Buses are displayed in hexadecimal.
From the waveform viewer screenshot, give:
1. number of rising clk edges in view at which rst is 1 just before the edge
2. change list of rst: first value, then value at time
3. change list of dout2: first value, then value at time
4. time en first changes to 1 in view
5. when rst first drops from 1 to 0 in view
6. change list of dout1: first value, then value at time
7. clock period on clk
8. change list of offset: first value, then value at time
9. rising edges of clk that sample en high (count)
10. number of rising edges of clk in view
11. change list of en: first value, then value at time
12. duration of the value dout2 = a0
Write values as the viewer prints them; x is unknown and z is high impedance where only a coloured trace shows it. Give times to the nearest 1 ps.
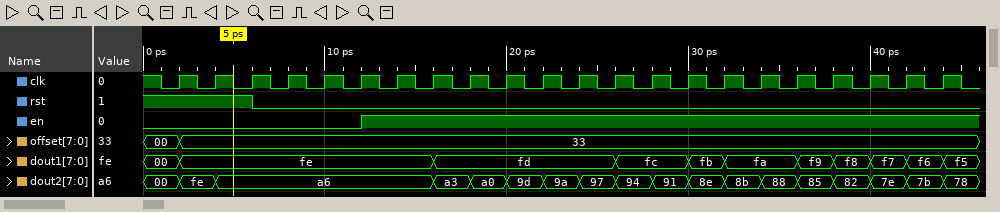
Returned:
3
1, 0 at 6 ps
00, fe at 2 ps, a6 at 4 ps, a3 at 16 ps, a0 at 18 ps, 9d at 20 ps, 9a at 22 ps, 97 at 24 ps, 94 at 26 ps, 91 at 28 ps, 8e at 30 ps, 8b at 32 ps, 88 at 34 ps, 85 at 36 ps, 82 at 38 ps, 7e at 40 ps, 7b at 42 ps, 78 at 44 ps
12 ps
6 ps
00, fe at 2 ps, fd at 16 ps, fc at 26 ps, fb at 30 ps, fa at 32 ps, f9 at 36 ps, f8 at 38 ps, f7 at 40 ps, f6 at 42 ps, f5 at 44 ps
2 ps
00, 33 at 2 ps
16
22
0, 1 at 12 ps
2 ps
